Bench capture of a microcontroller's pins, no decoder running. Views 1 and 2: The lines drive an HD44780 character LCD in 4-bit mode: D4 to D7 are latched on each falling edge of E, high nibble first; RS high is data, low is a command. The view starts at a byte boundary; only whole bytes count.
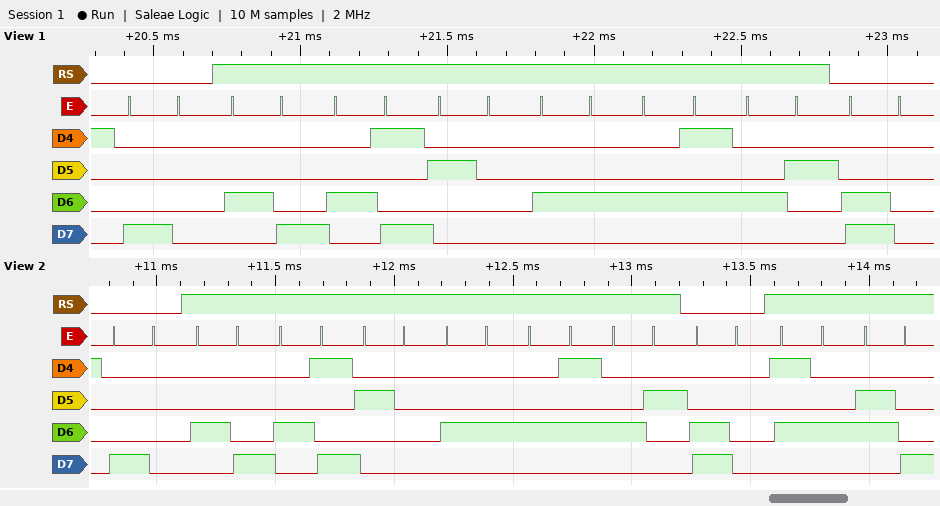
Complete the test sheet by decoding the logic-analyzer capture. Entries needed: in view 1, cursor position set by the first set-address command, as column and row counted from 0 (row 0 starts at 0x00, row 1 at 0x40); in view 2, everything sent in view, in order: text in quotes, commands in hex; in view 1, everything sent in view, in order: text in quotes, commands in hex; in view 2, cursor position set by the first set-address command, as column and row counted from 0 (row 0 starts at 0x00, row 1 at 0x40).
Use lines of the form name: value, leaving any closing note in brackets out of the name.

in view 1, cursor position set by the first set-address command, as column and row counted from 0: column 0, row 0
in view 2, everything sent in view, in order: text in quotes, commands in hex: 0x80 "HI DEB" 0xC0 "Th"
in view 1, everything sent in view, in order: text in quotes, commands in hex: 0x80 "HI DEB" 0xC0
in view 2, cursor position set by the first set-address command, as column and row counted from 0: column 0, row 0
